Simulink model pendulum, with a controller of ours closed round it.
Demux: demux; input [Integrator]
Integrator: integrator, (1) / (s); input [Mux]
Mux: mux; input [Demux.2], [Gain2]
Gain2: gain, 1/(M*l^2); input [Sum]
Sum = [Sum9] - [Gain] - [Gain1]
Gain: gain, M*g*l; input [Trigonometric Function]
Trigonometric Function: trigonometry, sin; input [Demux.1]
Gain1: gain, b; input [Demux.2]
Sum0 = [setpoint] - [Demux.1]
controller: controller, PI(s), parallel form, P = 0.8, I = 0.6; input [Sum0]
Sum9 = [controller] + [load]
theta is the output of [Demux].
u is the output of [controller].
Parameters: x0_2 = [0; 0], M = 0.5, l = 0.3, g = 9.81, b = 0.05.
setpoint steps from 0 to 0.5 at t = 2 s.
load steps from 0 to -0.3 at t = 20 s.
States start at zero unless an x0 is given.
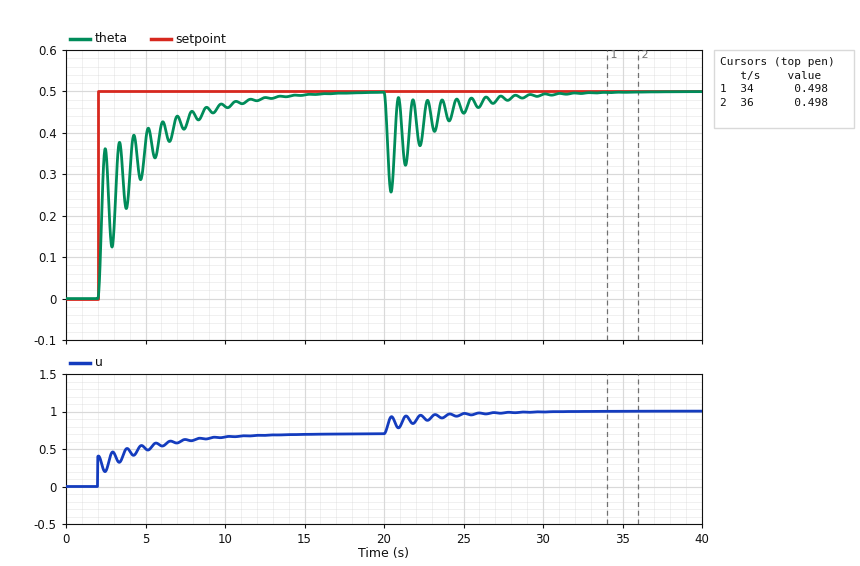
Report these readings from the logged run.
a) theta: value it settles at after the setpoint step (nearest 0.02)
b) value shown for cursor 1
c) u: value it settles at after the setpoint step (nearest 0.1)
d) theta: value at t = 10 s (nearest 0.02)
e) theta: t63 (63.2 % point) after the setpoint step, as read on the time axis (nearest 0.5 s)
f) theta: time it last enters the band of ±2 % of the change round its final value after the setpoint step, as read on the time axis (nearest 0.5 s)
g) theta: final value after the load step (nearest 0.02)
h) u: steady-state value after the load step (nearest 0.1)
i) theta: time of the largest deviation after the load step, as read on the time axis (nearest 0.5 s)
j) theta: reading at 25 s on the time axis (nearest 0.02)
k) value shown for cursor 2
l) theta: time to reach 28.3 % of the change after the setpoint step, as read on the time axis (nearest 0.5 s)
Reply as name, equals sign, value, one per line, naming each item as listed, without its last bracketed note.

theta: value it settles at after the setpoint step = 0.50
value shown for cursor 1 = 0.498
u: value it settles at after the setpoint step = 0.7
theta: value at t = 10 s = 0.46
theta: t63 (63.2 % point) after the setpoint step, as read on the time axis = 2.5 s
theta: time it last enters the band of ±2 % of the change round its final value after the setpoint step, as read on the time axis = 14.0 s
theta: final value after the load step = 0.50
u: steady-state value after the load step = 1.0
theta: time of the largest deviation after the load step, as read on the time axis = 20.5 s
theta: reading at 25 s on the time axis = 0.44
value shown for cursor 2 = 0.498
theta: time to reach 28.3 % of the change after the setpoint step, as read on the time axis = 2.0 s
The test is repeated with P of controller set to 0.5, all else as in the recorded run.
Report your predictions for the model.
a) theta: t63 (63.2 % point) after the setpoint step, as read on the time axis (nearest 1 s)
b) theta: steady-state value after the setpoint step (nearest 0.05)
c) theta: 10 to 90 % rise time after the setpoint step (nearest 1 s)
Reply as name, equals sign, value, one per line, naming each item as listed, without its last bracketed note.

theta: t63 (63.2 % point) after the setpoint step, as read on the time axis = 3 s
theta: steady-state value after the setpoint step = 0.50
theta: 10 to 90 % rise time after the setpoint step = 6 s
